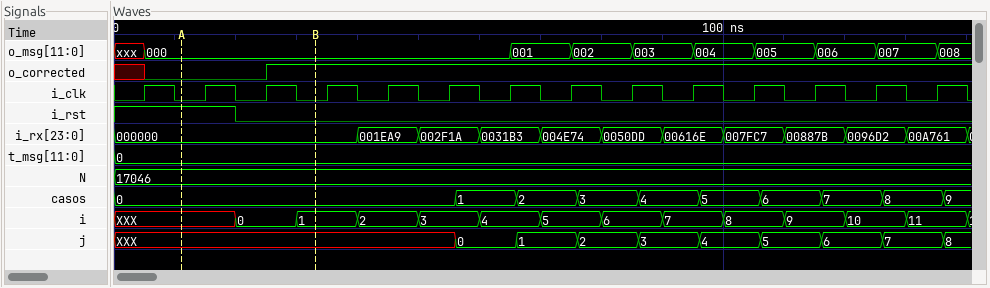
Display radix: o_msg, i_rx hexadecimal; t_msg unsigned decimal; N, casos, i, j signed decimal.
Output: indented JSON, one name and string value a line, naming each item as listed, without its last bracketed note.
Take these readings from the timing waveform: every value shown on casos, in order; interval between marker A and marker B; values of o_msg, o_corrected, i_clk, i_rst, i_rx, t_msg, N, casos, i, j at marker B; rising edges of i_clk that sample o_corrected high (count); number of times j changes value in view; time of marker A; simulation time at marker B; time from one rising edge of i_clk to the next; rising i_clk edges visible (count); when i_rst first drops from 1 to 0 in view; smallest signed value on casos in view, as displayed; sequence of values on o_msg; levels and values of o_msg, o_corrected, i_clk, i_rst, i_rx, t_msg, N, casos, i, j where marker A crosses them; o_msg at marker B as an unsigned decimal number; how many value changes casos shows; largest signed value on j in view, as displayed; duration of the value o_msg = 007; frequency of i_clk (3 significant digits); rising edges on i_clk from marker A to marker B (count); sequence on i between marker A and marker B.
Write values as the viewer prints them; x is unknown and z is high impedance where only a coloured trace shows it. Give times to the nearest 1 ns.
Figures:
{
  "every value shown on casos, in order": "0, 1, 2, 3, 4, 5, 6, 7, 8, 9",
  "interval between marker A and marker B": "22 ns",
  "values of o_msg, o_corrected, i_clk, i_rst, i_rx, t_msg, N, casos, i, j at marker B": "o_msg=000, o_corrected=1, i_clk=0, i_rst=0, i_rx=000000, t_msg=0, N=17046, casos=0, i=1, j=XXX",
  "rising edges of i_clk that sample o_corrected high": "11",
  "number of times j changes value in view": "9",
  "time of marker A": "11 ns",
  "simulation time at marker B": "33 ns",
  "time from one rising edge of i_clk to the next": "10 ns",
  "rising i_clk edges visible": "14",
  "when i_rst first drops from 1 to 0 in view": "20 ns",
  "smallest signed value on casos in view, as displayed": "0",
  "sequence of values on o_msg": "xxx, 000, 001, 002, 003, 004, 005, 006, 007, 008",
  "levels and values of o_msg, o_corrected, i_clk, i_rst, i_rx, t_msg, N, casos, i, j where marker A crosses them": "o_msg=000, o_corrected=0, i_clk=0, i_rst=1, i_rx=000000, t_msg=0, N=17046, casos=0, i=XXX, j=XXX",
  "o_msg at marker B as an unsigned decimal number": "0",
  "how many value changes casos shows": "9",
  "largest signed value on j in view, as displayed": "8",
  "duration of the value o_msg = 007": "10 ns",
  "frequency of i_clk": "100 MHz",
  "rising edges on i_clk from marker A to marker B": "2",
  "sequence on i between marker A and marker B": "XXX, 0, 1"
}
